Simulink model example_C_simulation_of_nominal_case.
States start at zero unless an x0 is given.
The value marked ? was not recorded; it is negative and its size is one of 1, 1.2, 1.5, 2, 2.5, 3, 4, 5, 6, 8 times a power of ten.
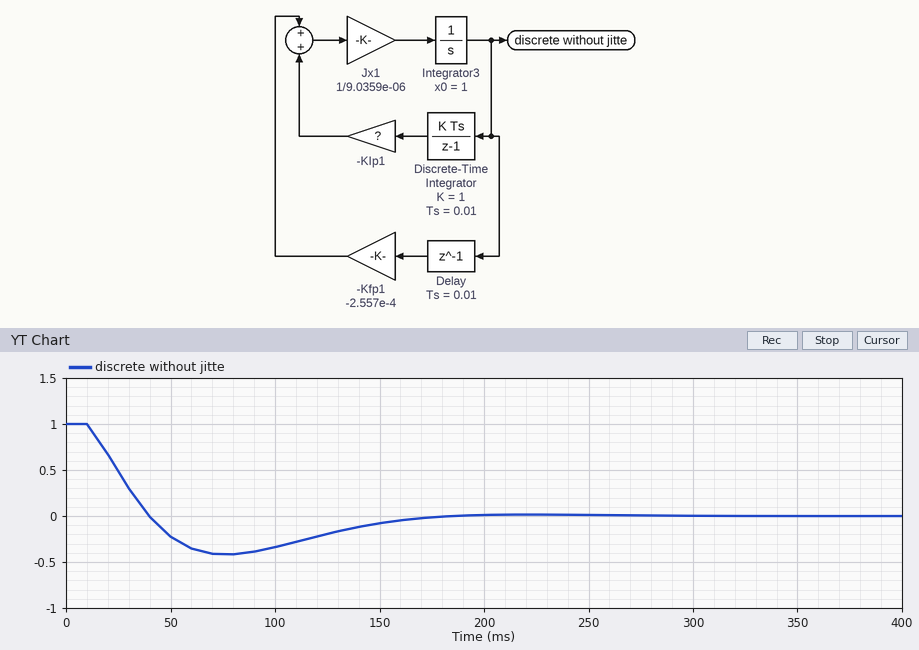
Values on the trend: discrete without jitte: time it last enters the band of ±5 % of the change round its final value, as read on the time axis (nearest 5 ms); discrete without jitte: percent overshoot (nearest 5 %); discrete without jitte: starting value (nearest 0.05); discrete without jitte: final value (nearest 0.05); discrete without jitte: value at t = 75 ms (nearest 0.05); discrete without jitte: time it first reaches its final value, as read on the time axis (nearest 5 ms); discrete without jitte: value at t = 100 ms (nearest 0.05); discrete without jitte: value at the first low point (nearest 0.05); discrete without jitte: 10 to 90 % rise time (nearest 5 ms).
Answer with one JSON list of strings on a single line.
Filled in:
["160 ms", "40 %", "1.00", "0.00", "-0.40", "40 ms", "-0.35", "-0.40", "25 ms"]
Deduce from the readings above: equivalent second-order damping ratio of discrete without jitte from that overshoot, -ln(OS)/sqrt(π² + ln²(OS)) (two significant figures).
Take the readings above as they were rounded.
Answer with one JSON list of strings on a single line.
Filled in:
["0.28"]
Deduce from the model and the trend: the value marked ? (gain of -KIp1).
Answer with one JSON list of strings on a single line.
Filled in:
["-0.004"]
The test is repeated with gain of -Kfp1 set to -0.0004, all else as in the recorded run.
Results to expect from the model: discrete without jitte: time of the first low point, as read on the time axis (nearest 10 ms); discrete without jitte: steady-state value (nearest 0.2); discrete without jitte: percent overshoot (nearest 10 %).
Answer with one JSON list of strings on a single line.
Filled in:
["50 ms", "0.0", "50 %"]
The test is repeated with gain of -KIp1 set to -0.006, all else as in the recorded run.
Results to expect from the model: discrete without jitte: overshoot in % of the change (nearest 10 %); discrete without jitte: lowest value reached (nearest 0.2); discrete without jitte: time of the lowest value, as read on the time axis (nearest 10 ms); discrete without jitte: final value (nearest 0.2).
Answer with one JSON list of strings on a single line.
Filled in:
["60 %", "-0.6", "70 ms", "0.0"]
